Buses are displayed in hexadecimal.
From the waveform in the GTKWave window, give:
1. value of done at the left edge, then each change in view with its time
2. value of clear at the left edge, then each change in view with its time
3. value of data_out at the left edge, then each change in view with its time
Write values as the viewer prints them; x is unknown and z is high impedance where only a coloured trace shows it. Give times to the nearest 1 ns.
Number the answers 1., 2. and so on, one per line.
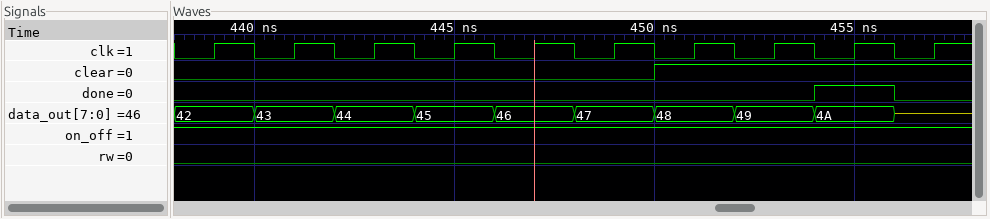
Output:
1. 0, 1 at 454 ns, 0 at 456 ns
2. 0, 1 at 450 ns
3. 42, 43 at 440 ns, 44 at 442 ns, 45 at 444 ns, 46 at 446 ns, 47 at 448 ns, 48 at 450 ns, 49 at 452 ns, 4A at 454 ns, z at 456 ns
